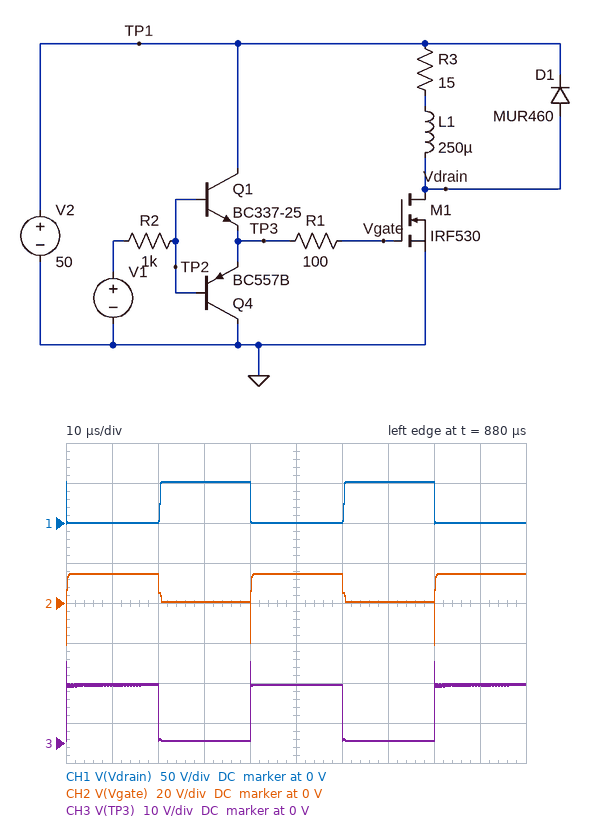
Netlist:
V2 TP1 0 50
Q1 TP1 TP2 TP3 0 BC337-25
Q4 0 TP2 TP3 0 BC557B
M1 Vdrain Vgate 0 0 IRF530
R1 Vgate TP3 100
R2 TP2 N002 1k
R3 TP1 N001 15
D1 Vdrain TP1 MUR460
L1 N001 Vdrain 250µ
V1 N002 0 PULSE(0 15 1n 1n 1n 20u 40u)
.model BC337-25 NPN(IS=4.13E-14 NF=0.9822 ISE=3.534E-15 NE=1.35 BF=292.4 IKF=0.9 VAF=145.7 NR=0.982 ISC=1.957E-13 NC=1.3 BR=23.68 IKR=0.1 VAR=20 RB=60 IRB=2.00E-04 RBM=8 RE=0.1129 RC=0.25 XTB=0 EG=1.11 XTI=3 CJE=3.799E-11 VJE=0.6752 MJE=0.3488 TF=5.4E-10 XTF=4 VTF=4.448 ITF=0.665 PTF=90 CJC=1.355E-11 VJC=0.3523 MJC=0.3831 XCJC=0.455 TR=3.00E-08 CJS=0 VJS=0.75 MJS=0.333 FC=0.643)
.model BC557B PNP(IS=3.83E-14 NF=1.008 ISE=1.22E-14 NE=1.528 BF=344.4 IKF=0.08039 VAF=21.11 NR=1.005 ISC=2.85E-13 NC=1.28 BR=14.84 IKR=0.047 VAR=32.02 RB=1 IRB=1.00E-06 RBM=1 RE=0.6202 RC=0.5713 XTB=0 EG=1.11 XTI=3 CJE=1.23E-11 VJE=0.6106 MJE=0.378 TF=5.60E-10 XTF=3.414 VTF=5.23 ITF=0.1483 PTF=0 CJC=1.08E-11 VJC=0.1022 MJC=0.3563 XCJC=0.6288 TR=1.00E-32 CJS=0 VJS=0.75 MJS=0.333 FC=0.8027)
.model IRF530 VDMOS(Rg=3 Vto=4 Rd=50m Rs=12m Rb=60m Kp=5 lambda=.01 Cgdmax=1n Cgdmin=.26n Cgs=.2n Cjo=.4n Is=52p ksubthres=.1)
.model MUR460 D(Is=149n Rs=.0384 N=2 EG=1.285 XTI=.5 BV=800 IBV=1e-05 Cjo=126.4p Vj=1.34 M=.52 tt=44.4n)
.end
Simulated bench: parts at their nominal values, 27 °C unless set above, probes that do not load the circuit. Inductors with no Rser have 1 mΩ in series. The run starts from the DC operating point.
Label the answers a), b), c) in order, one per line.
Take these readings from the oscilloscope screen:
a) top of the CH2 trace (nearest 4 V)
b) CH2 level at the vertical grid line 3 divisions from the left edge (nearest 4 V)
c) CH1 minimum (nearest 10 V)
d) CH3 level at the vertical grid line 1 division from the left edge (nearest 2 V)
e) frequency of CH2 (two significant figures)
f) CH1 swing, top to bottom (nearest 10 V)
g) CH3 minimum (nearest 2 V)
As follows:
a) 16 V
b) 0 V
c) 0 V
d) 14 V
e) 25 kHz
f) 50 V
g) 0 V
